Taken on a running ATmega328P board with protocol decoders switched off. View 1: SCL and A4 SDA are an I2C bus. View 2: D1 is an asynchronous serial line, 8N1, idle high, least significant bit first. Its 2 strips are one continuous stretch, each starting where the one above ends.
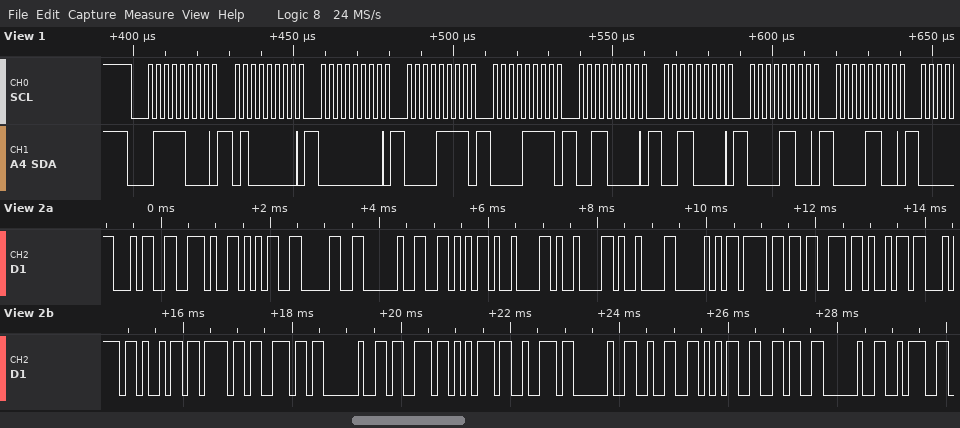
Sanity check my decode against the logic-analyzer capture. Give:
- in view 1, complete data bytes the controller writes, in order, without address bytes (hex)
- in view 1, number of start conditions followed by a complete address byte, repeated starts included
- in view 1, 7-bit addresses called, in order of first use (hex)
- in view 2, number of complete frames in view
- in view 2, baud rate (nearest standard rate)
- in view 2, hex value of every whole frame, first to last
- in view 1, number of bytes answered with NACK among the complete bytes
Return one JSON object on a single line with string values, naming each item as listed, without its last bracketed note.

{"in view 1, complete data bytes the controller writes, in order, without address bytes": "40 00 0F 0F 30 30 0C 0C", "in view 1, number of start conditions followed by a complete address byte, repeated starts included": "1", "in view 1, 7-bit addresses called, in order of first use": "0x3C", "in view 2, number of complete frames in view": "27", "in view 2, baud rate": "9600 baud", "in view 2, hex value of every whole frame, first to last": "0x34 0x2E 0x35 0x30 0x20 0x56 0x09 0x09 0x09 0x50 0x6F 0x73 0x69 0x74 0x69 0x6F 0x6E 0x20 0x73 0x75 0x72 0x20 0x32 0x35 0x36 0x20 0x3A", "in view 1, number of bytes answered with NACK among the complete bytes": "0"}
